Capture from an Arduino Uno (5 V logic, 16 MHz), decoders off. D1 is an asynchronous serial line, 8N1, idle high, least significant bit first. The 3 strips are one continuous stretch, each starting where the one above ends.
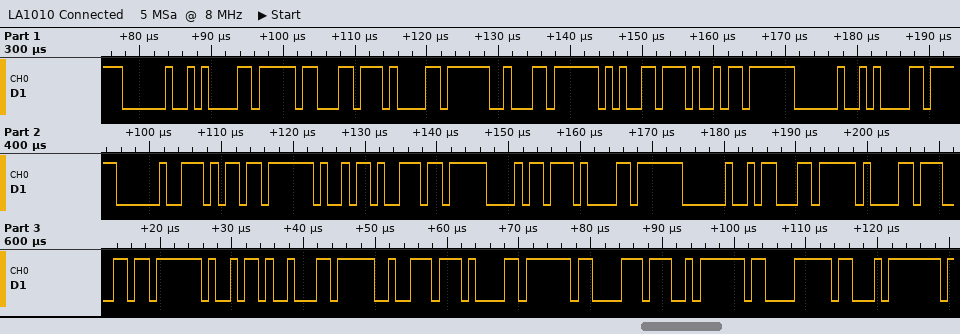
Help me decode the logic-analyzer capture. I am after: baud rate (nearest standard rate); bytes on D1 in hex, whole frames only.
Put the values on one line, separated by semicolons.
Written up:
1000000 baud; 20 61 63 61 62 65 69 20 61 20 6D 69 6E 68 61 20 63 61 6C 69 62 72 61 C3 A7 C3 A3
